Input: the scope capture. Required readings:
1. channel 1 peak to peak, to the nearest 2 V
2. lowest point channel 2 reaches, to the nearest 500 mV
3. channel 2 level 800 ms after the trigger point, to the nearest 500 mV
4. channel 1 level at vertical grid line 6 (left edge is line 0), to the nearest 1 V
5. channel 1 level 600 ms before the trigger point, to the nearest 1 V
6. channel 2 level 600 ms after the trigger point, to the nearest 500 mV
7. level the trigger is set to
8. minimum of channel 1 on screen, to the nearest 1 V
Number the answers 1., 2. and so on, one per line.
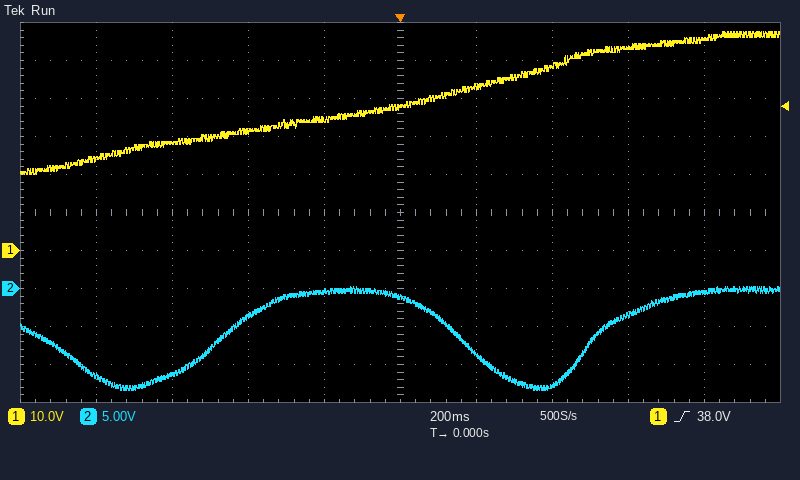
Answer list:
1. 38 V
2. -13.5 V
3. -500 mV
4. 43 V
5. 28 V
6. -3.5 V
7. 38.0 V
8. 20 V
